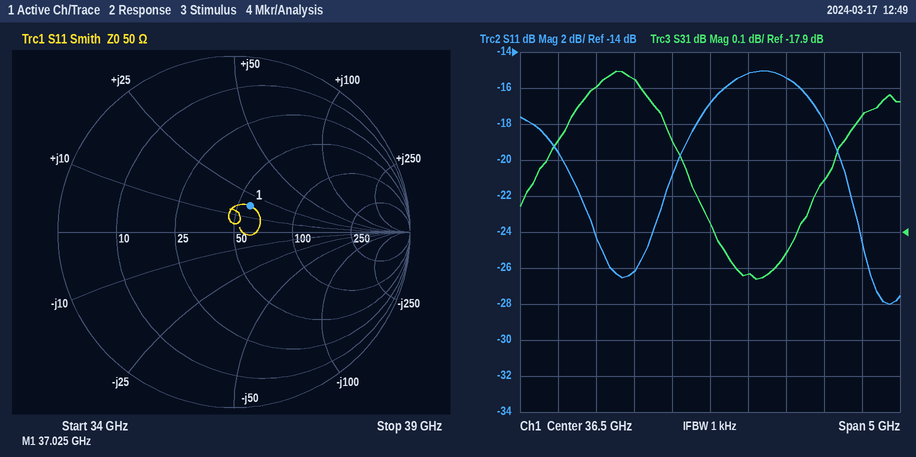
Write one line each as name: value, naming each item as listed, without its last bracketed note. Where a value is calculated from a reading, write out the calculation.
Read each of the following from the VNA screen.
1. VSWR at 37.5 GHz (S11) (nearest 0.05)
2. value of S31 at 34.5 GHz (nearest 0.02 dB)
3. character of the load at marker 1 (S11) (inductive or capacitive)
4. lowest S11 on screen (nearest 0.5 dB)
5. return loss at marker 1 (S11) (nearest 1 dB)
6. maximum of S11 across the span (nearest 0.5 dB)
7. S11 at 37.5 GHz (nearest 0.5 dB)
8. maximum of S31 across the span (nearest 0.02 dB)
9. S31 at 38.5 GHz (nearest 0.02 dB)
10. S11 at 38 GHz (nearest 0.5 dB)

VSWR at 37.5 GHz (S11): |Γ| = 10^(-15.5/20) = 0.1679; VSWR = (1 + 0.1679)/(1 − 0.1679) ≈ 1.40
value of S31 at 34.5 GHz: -17.64 dB
character of the load at marker 1 (S11): inductive
lowest S11 on screen: -28.0 dB
return loss at marker 1 (S11): 15 dB
maximum of S11 across the span: -15.0 dB
S11 at 37.5 GHz: -15.5 dB
maximum of S31 across the span: -17.46 dB
S31 at 38.5 GHz: -17.58 dB
S11 at 38 GHz: -18.0 dB
